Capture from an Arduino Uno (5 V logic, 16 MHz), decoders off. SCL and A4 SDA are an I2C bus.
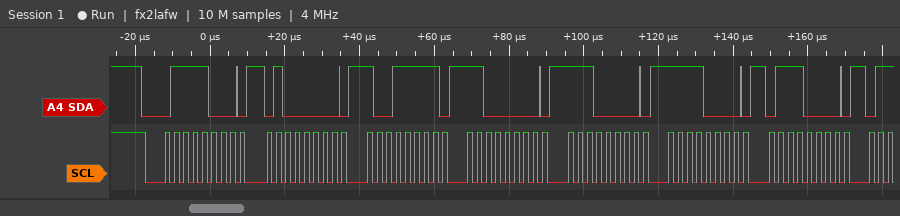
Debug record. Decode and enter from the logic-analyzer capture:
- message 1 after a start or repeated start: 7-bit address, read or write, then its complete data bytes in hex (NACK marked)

0x3C write: 40 9F C0 E0 F0 70
